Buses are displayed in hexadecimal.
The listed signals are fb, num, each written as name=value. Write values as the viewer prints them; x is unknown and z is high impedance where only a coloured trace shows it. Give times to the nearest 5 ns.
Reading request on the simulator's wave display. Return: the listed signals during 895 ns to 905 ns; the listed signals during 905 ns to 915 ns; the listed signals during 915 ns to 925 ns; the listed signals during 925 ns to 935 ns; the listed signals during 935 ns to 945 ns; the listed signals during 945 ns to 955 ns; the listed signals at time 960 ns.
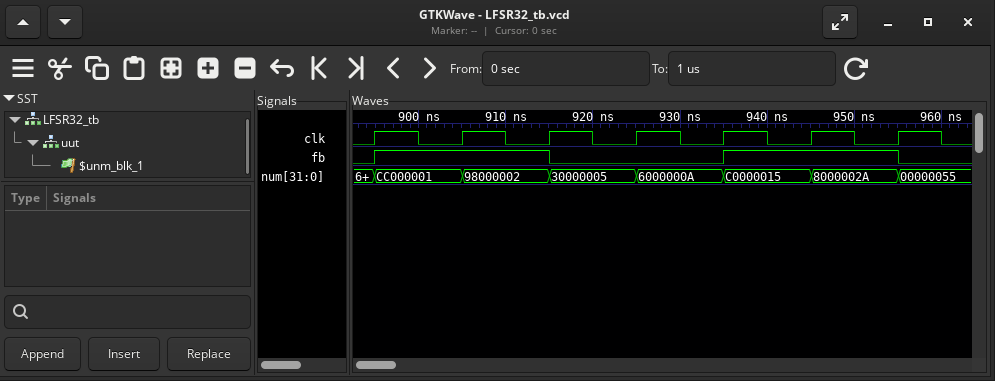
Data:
fb=1, num=CC000001
fb=1, num=98000002
fb=0, num=30000005
fb=0, num=6000000A
fb=1, num=C0000015
fb=1, num=8000002A
fb=0, num=00000055
